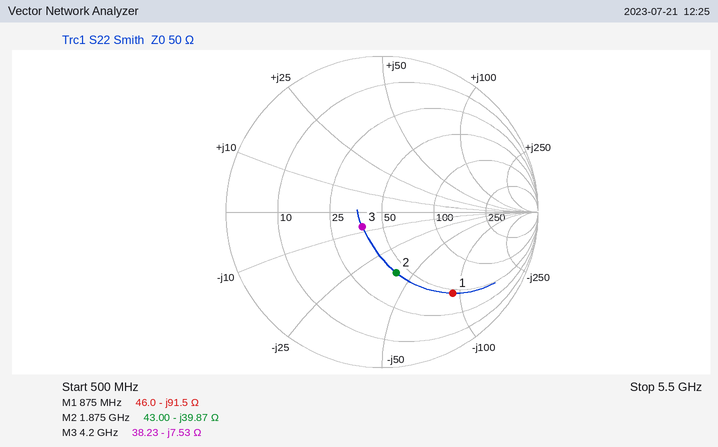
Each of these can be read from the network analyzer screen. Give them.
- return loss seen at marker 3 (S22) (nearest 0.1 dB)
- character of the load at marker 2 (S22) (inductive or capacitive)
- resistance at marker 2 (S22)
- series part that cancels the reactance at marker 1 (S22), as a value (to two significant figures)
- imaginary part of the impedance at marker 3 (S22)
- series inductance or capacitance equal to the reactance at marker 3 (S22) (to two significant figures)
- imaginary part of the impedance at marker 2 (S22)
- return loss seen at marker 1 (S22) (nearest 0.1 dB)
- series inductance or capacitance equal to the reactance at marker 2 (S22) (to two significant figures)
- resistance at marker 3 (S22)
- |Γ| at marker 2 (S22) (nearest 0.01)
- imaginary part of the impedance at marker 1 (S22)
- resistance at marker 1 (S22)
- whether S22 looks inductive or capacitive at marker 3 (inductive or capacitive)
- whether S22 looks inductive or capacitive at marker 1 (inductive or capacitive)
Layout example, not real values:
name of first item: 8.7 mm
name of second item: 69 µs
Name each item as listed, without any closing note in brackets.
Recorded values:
return loss seen at marker 3 (S22): 16.0 dB
character of the load at marker 2 (S22): capacitive
resistance at marker 2: 43.00 Ω
series part that cancels the reactance at marker 1 (S22), as a value: 17 nH
imaginary part of the impedance at marker 3: -7.53 Ω
series inductance or capacitance equal to the reactance at marker 3 (S22): 5.0 pF
imaginary part of the impedance at marker 2: -39.87 Ω
return loss seen at marker 1 (S22): 3.2 dB
series inductance or capacitance equal to the reactance at marker 2 (S22): 2.1 pF
resistance at marker 3: 38.23 Ω
|Γ| at marker 2 (S22): 0.40
imaginary part of the impedance at marker 1: -91.5 Ω
resistance at marker 1: 46.0 Ω
whether S22 looks inductive or capacitive at marker 3: capacitive
whether S22 looks inductive or capacitive at marker 1: capacitive
